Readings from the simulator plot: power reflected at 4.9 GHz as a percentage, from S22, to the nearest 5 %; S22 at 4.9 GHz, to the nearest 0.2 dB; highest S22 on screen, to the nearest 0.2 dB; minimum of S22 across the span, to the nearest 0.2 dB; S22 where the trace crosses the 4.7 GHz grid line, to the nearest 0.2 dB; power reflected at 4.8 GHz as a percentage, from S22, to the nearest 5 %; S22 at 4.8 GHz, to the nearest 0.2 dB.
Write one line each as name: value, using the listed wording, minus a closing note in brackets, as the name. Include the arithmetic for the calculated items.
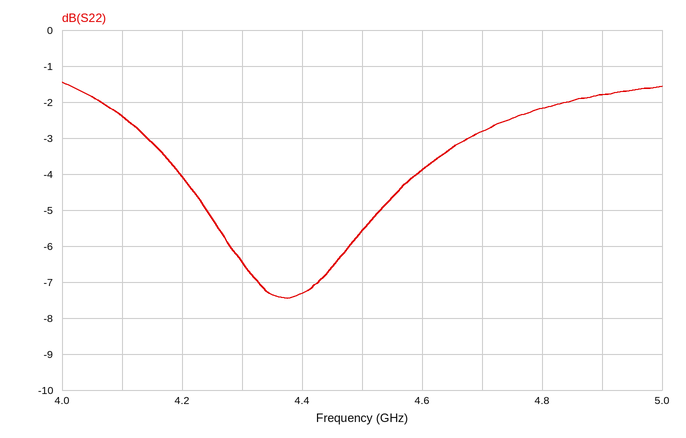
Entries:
power reflected at 4.9 GHz as a percentage, from S22, to the nearest 5 %: 10^(-1.8/10) ≈ 66.1 %, so 65 % to the nearest 5 %
S22 at 4.9 GHz, to the nearest 0.2 dB: -1.8 dB
highest S22 on screen, to the nearest 0.2 dB: -1.4 dB
minimum of S22 across the span, to the nearest 0.2 dB: -7.4 dB
S22 where the trace crosses the 4.7 GHz grid line, to the nearest 0.2 dB: -2.8 dB
power reflected at 4.8 GHz as a percentage, from S22, to the nearest 5 %: 10^(-2.2/10) ≈ 60 %
S22 at 4.8 GHz, to the nearest 0.2 dB: -2.2 dB
